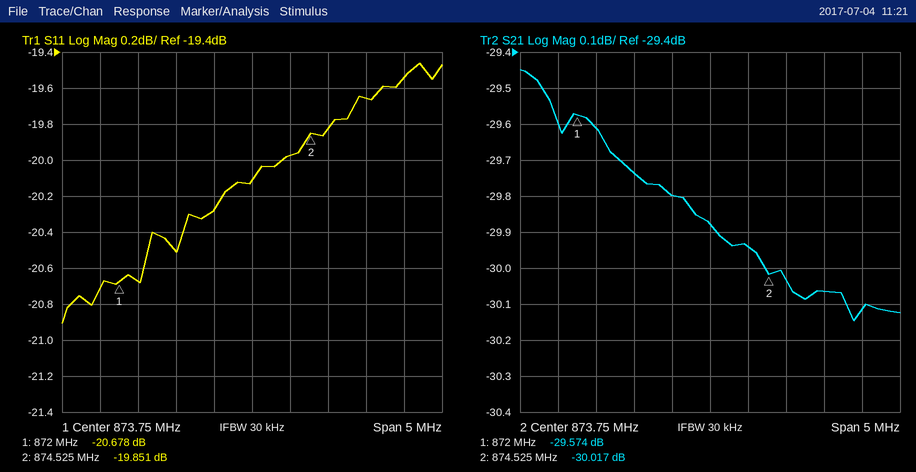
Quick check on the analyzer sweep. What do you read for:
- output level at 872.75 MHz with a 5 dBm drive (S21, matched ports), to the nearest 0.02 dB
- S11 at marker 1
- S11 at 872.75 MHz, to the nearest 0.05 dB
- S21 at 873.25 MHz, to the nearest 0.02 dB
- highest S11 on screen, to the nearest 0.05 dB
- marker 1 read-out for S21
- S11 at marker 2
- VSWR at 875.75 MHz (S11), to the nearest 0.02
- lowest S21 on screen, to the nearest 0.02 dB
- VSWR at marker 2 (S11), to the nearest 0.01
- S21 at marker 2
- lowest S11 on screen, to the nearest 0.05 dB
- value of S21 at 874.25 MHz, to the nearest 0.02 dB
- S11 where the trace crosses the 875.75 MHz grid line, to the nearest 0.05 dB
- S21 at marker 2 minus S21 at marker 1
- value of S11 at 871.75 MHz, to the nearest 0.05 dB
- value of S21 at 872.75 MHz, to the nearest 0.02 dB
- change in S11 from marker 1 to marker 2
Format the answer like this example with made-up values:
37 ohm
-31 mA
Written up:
-24.74 dBm
-20.678 dB
-20.50 dB
-29.80 dB
-19.45 dB
-29.574 dB
-19.851 dB
1.24
-30.14 dB
1.23
-30.017 dB
-20.90 dB
-29.94 dB
-19.55 dB
-0.443 dB
-20.70 dB
-29.74 dB
0.827 dB
